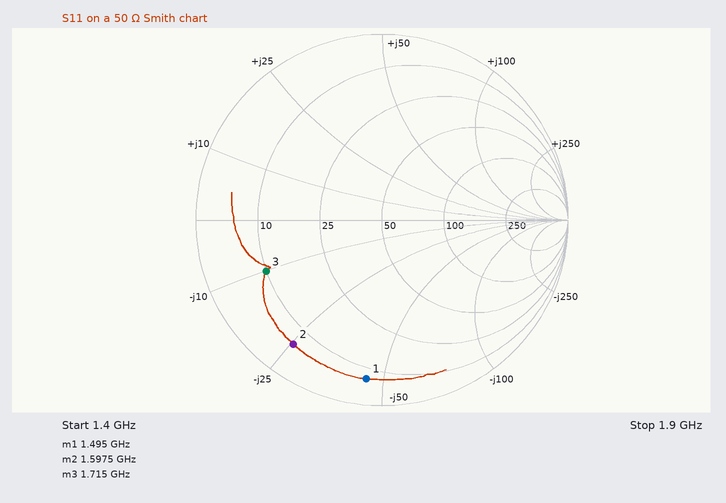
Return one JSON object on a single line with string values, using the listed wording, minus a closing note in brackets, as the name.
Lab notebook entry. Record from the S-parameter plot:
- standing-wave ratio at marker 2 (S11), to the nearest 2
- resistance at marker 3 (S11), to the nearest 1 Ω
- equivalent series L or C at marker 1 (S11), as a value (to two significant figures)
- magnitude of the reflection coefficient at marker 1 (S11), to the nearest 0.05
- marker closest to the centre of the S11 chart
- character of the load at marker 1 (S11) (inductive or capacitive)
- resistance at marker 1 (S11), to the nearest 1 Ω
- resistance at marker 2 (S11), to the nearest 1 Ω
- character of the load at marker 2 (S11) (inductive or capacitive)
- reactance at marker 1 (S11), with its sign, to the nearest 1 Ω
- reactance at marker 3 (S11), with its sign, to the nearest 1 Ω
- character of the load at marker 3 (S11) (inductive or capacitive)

{"standing-wave ratio at marker 2 (S11), to the nearest 2": "10", "resistance at marker 3 (S11), to the nearest 1 Ω": "10 Ω", "equivalent series L or C at marker 1 (S11), as a value": "2.4 pF", "magnitude of the reflection coefficient at marker 1 (S11), to the nearest 0.05": "0.85", "marker closest to the centre of the S11 chart": "marker 3", "character of the load at marker 1 (S11)": "capacitive", "resistance at marker 1 (S11), to the nearest 1 Ω": "7 Ω", "resistance at marker 2 (S11), to the nearest 1 Ω": "6 Ω", "character of the load at marker 2 (S11)": "capacitive", "reactance at marker 1 (S11), with its sign, to the nearest 1 Ω": "-45 Ω", "reactance at marker 3 (S11), with its sign, to the nearest 1 Ω": "-10 Ω", "character of the load at marker 3 (S11)": "capacitive"}
